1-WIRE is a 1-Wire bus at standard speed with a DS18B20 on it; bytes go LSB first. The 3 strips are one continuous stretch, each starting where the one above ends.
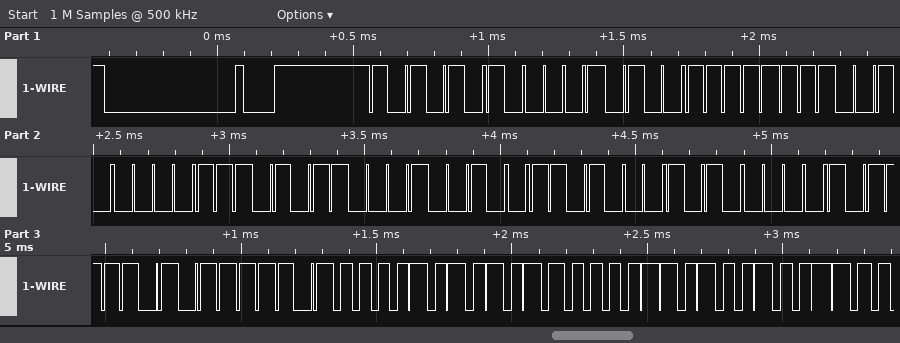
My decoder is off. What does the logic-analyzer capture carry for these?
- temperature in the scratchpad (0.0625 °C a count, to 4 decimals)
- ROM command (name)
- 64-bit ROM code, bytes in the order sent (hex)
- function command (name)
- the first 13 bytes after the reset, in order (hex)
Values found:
85.0000 °C
Match ROM
28 FF 04 D7 48 16 05 BD
Read Scratchpad
55 28 FF 04 D7 48 16 05 BD BE 50 05 4B
